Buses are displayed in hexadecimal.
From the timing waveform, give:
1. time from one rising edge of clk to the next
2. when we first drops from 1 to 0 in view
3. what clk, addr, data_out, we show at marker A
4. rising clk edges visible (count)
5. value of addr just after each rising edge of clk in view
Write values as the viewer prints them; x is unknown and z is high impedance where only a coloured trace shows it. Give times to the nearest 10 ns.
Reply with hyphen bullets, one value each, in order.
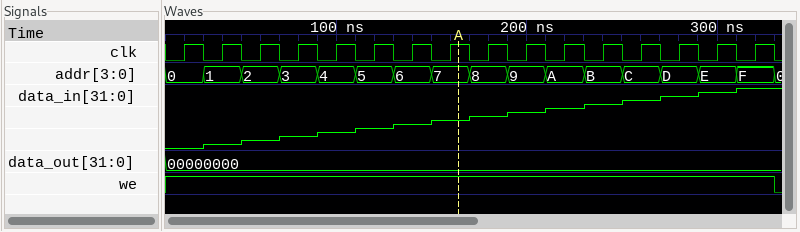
- 20 ns
- 330 ns
- clk=1, addr=7, data_out=00000000, we=1
- 16
- 0, 1, 2, 3, 4, 5, 6, 7, 8, 9, A, B, C, D, E, F
